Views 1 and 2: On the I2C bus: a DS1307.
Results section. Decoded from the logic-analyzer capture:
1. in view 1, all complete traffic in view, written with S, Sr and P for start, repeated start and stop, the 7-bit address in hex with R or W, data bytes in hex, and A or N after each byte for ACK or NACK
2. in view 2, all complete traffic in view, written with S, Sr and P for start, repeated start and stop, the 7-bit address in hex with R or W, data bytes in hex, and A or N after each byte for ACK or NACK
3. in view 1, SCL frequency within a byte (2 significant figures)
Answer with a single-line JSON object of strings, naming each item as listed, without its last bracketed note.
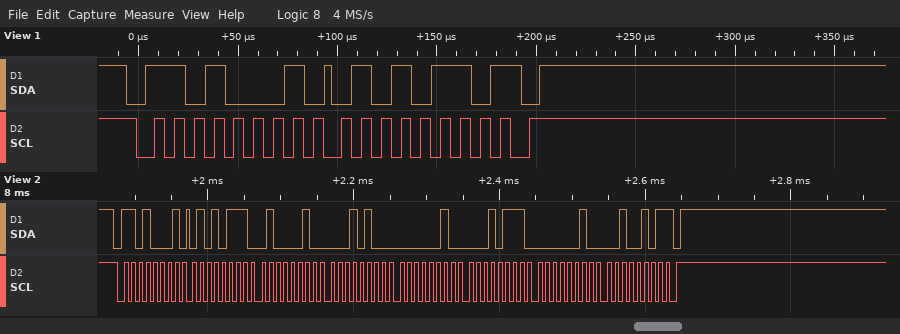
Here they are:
{"in view 1, all complete traffic in view, written with S, Sr and P for start, repeated start and stop, the 7-bit address in hex with R or W, data bytes in hex, and A or N after each byte for ACK or NACK": "S 68R A 56 N P", "in view 2, all complete traffic in view, written with S, Sr and P for start, repeated start and stop, the 7-bit address in hex with R or W, data bytes in hex, and A or N after each byte for ACK or NACK": "S 68R A 57 A 42 A 14 A 02 A 17 A 02 A 25 N P", "in view 1, SCL frequency within a byte": "100 kHz"}
